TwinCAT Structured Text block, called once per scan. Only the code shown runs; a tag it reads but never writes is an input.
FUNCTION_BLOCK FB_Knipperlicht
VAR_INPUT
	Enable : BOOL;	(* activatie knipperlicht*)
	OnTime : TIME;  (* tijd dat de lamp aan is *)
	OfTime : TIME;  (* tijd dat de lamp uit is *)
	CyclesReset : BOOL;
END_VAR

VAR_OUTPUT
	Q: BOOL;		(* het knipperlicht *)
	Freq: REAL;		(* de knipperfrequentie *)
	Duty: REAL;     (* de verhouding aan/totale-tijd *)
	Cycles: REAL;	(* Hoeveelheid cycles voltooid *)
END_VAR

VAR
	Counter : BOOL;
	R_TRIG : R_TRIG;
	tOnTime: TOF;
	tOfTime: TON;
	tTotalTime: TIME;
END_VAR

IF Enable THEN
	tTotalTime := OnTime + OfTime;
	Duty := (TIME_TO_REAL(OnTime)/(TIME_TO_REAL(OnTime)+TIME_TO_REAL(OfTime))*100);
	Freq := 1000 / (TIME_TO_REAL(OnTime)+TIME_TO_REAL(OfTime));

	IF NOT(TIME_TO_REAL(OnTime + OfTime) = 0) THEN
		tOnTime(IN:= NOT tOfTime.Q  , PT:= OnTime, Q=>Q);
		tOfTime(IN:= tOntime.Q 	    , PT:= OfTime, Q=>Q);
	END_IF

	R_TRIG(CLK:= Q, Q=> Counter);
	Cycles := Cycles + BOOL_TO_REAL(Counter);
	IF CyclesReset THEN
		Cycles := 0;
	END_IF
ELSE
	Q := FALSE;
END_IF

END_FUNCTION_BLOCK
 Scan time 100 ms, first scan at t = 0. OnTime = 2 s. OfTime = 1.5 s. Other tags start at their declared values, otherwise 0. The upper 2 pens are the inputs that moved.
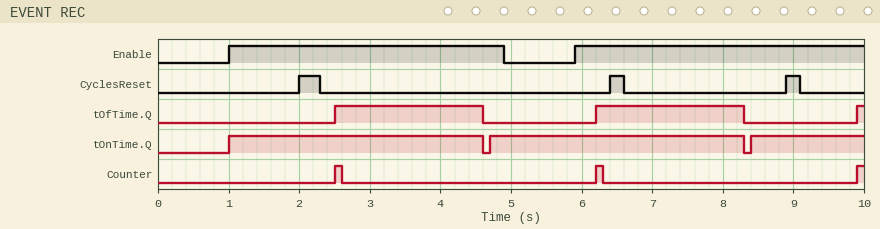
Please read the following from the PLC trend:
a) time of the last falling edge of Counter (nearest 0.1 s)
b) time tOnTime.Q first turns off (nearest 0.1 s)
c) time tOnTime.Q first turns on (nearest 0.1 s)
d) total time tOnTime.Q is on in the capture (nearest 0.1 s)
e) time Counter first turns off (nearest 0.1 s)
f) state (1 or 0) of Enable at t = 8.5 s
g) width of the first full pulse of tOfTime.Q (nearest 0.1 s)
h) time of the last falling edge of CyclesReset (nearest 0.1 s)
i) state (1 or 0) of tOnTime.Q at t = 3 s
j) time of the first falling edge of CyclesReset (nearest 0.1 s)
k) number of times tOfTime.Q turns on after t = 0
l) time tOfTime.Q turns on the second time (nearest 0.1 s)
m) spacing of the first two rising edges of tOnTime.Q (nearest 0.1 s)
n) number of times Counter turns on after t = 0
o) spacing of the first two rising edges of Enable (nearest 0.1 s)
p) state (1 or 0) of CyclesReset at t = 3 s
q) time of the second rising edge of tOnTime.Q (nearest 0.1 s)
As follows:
6.3 s
4.6 s
1.0 s
8.8 s
2.6 s
1
2.1 s
9.1 s
1
2.3 s
3
6.2 s
3.7 s
3
4.9 s
0
4.7 s
